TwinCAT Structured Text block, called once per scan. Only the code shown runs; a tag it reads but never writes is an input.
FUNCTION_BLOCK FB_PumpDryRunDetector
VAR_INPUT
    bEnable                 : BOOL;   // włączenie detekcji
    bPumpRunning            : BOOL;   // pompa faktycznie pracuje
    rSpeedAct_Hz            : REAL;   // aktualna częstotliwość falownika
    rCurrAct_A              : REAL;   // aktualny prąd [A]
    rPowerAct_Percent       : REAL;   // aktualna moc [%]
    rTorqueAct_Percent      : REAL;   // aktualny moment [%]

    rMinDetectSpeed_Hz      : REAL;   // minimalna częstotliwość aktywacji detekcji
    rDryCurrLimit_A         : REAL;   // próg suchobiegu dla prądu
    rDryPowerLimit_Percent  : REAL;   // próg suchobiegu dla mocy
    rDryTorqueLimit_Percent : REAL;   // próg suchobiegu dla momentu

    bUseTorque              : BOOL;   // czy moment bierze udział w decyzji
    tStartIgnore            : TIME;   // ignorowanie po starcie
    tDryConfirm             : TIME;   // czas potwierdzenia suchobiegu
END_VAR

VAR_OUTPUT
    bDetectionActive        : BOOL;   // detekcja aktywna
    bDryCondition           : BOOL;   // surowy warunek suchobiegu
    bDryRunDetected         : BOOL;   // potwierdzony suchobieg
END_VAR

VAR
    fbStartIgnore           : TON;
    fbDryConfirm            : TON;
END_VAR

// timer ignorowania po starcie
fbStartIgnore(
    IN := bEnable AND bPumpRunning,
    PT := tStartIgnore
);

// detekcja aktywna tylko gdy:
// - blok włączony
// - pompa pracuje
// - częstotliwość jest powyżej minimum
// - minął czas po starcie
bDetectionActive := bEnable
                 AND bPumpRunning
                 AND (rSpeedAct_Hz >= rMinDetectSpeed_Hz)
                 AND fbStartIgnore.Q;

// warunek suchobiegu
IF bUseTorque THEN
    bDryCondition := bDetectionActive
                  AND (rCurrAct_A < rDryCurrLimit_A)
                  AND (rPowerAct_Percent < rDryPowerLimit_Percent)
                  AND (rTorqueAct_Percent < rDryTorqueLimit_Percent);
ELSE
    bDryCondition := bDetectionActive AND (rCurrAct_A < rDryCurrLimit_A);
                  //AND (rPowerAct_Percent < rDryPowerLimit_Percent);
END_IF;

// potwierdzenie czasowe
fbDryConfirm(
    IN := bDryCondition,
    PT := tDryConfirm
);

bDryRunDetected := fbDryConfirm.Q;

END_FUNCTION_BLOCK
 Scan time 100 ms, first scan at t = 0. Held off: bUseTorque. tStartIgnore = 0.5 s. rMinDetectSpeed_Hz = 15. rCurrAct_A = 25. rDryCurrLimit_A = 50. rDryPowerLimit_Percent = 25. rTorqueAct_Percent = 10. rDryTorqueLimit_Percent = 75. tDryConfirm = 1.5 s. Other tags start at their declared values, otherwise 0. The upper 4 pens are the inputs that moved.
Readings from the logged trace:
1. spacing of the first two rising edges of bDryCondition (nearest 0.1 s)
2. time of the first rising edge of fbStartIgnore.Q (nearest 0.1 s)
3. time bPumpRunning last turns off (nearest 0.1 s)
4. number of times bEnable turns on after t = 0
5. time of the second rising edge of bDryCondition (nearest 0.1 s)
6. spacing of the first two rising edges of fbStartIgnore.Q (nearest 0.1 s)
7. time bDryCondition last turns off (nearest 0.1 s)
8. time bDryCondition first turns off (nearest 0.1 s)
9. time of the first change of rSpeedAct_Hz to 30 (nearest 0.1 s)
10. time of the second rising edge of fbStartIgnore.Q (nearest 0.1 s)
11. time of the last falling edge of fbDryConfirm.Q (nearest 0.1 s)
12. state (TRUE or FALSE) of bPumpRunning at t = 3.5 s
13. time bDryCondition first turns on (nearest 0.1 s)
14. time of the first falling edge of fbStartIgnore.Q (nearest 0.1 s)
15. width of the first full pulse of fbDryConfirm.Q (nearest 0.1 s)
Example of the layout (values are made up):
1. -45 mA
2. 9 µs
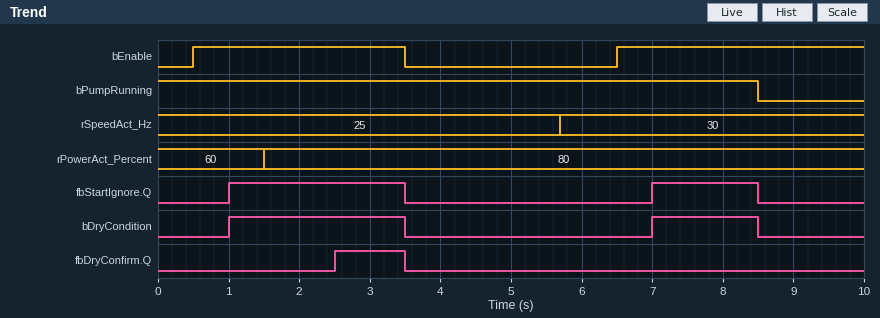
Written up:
1. 6.0 s
2. 1.0 s
3. 8.5 s
4. 2
5. 7.0 s
6. 6.0 s
7. 8.5 s
8. 3.5 s
9. 5.7 s
10. 7.0 s
11. 3.5 s
12. TRUE
13. 1.0 s
14. 3.5 s
15. 1.0 s
